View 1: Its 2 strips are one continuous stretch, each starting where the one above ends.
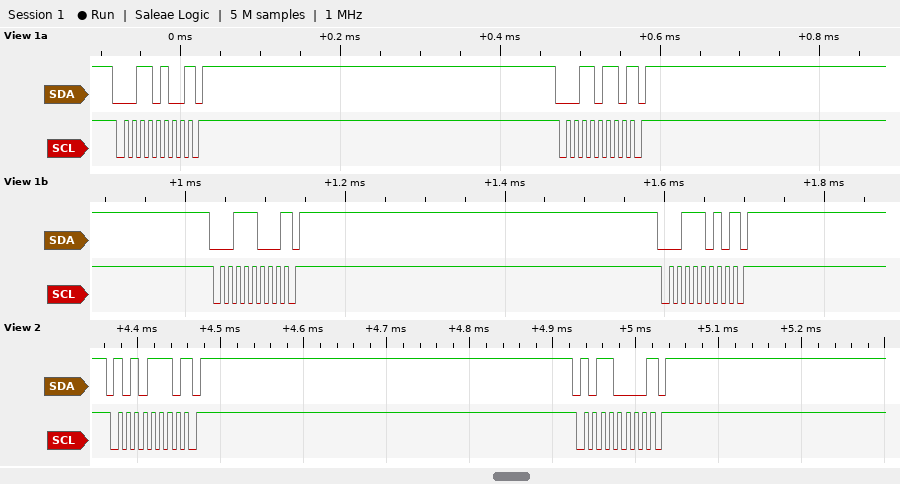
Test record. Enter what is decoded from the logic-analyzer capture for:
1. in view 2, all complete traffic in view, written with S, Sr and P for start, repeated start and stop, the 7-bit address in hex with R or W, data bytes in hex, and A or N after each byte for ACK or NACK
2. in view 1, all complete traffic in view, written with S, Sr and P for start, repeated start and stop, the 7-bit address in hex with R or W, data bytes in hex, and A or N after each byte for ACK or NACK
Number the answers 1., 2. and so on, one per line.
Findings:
1. S 57W N P S 58W N P
2. S 1AW N P S 1BW N P S 1CW N P S 1DW N P
